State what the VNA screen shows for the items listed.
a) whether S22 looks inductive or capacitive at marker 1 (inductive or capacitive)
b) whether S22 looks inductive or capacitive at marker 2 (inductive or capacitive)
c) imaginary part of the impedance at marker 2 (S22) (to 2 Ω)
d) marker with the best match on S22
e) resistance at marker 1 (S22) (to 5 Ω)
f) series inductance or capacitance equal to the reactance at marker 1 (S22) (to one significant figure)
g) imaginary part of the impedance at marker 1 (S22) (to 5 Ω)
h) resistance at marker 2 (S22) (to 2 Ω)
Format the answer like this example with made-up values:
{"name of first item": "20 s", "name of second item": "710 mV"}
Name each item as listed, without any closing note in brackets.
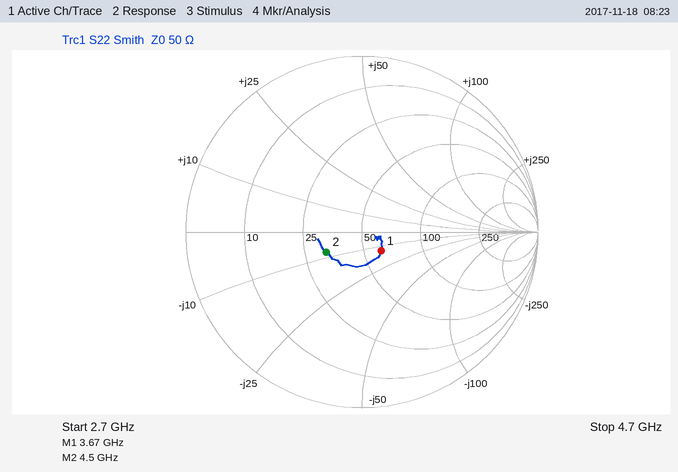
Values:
{"whether S22 looks inductive or capacitive at marker 1": "capacitive", "whether S22 looks inductive or capacitive at marker 2": "capacitive", "imaginary part of the impedance at marker 2 (S22)": "-8 Ω", "marker with the best match on S22": "marker 1", "resistance at marker 1 (S22)": "60 Ω", "series inductance or capacitance equal to the reactance at marker 1 (S22)": "3 pF", "imaginary part of the impedance at marker 1 (S22)": "-15 Ω", "resistance at marker 2 (S22)": "32 Ω"}
